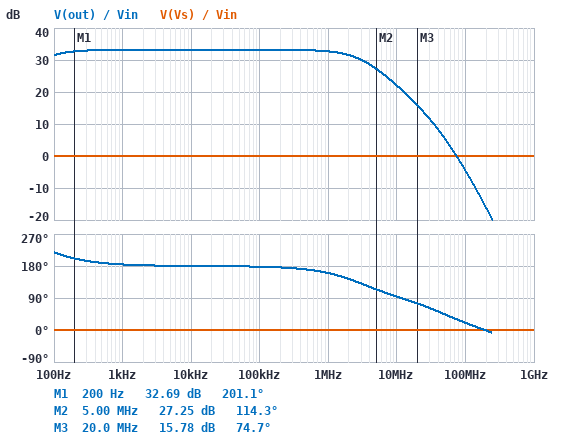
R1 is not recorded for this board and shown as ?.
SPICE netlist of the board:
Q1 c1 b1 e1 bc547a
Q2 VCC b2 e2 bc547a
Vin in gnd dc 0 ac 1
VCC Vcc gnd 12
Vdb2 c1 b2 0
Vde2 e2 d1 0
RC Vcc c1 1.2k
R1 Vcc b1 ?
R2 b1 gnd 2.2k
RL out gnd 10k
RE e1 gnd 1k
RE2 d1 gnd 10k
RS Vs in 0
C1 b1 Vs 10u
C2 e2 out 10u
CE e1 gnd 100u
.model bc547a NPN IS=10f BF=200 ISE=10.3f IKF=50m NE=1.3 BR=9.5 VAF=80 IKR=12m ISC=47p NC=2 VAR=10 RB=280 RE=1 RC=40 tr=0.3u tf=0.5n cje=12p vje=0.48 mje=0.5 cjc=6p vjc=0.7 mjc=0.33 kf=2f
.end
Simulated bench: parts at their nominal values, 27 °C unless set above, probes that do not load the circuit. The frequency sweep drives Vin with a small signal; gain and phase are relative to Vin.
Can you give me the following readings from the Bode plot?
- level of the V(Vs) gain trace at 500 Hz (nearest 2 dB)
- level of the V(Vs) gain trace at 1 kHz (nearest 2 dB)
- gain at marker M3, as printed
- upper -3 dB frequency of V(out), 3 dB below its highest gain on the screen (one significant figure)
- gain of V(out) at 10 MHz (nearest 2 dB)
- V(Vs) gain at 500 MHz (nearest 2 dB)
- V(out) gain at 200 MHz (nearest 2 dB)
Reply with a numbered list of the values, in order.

1. 0 dB
2. 0 dB
3. 15.78 dB
4. 3 MHz
5. 22 dB
6. 0 dB
7. -16 dB
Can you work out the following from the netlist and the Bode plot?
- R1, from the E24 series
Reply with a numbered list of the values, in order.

1. 12 kΩ
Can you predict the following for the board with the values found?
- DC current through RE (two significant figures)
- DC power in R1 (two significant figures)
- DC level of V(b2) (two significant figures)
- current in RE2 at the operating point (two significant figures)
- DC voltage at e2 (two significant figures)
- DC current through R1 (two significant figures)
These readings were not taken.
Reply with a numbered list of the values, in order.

1. 1.2 mA
2. 8.6 mW
3. 11 V
4. 990 µA
5. 9.9 V
6. 850 µA
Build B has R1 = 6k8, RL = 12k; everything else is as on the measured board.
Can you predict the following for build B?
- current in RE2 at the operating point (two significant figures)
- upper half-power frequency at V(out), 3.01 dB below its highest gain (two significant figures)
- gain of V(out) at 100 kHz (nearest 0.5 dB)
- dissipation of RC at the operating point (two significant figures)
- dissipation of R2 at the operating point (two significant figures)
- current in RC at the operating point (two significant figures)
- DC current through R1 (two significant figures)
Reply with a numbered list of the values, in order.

1. 870 µA
2. 1.9 MHz
3. 37.5 dB
4. 5.9 mW
5. 3.8 mW
6. 2.2 mA
7. 1.3 mA
